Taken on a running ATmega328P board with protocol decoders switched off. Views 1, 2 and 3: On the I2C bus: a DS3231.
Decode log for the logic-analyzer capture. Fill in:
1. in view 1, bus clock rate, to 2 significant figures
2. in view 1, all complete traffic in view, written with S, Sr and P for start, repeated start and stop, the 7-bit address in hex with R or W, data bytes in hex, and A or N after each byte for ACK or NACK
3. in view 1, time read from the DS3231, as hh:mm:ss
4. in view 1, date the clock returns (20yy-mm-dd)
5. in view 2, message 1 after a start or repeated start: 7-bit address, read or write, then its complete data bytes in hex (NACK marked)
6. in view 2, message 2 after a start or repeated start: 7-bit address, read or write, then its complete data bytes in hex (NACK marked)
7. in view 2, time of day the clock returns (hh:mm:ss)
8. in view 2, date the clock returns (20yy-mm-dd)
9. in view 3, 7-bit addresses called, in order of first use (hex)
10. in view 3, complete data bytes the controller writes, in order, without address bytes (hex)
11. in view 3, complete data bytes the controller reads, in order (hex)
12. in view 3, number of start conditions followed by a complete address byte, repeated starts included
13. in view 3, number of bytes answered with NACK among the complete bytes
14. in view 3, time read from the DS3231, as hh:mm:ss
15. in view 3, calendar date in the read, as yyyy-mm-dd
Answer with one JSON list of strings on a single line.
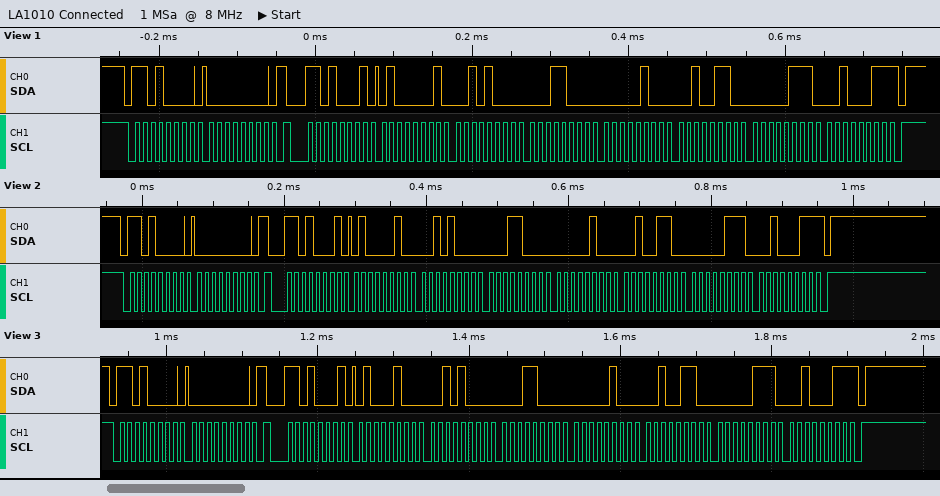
["100 kHz", "S 68W A 00 A Sr 68R A 41 A 28 A 18 A 04 A 26 A 07 A 23 N P", "18:28:41", "2023-07-26", "0x68 write: 00", "0x68 read: 42 28 18 04 26 07 23 NACK", "18:28:42", "2023-07-26", "0x68", "00", "44 28 18 04 26 07 23", "2", "1", "18:28:44", "2023-07-26"]
